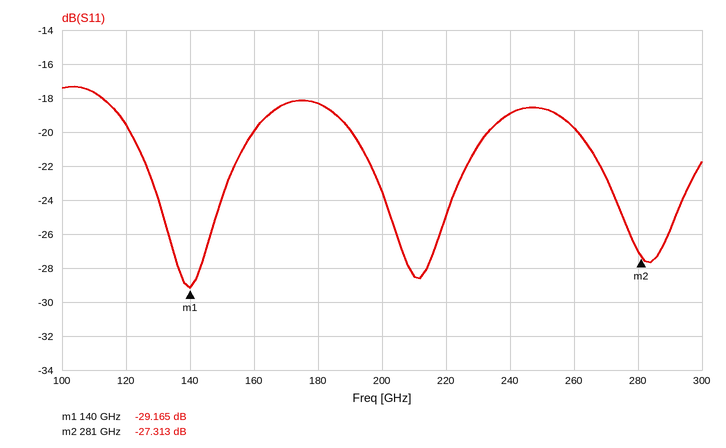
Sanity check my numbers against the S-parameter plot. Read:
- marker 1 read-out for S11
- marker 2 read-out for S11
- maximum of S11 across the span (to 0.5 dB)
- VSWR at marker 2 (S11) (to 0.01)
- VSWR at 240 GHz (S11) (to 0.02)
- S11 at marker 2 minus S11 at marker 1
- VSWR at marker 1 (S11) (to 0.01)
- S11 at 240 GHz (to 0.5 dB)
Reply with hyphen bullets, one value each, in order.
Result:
- -29.165 dB
- -27.313 dB
- -17.5 dB
- 1.09
- 1.26
- 1.852 dB
- 1.07
- -19.0 dB
